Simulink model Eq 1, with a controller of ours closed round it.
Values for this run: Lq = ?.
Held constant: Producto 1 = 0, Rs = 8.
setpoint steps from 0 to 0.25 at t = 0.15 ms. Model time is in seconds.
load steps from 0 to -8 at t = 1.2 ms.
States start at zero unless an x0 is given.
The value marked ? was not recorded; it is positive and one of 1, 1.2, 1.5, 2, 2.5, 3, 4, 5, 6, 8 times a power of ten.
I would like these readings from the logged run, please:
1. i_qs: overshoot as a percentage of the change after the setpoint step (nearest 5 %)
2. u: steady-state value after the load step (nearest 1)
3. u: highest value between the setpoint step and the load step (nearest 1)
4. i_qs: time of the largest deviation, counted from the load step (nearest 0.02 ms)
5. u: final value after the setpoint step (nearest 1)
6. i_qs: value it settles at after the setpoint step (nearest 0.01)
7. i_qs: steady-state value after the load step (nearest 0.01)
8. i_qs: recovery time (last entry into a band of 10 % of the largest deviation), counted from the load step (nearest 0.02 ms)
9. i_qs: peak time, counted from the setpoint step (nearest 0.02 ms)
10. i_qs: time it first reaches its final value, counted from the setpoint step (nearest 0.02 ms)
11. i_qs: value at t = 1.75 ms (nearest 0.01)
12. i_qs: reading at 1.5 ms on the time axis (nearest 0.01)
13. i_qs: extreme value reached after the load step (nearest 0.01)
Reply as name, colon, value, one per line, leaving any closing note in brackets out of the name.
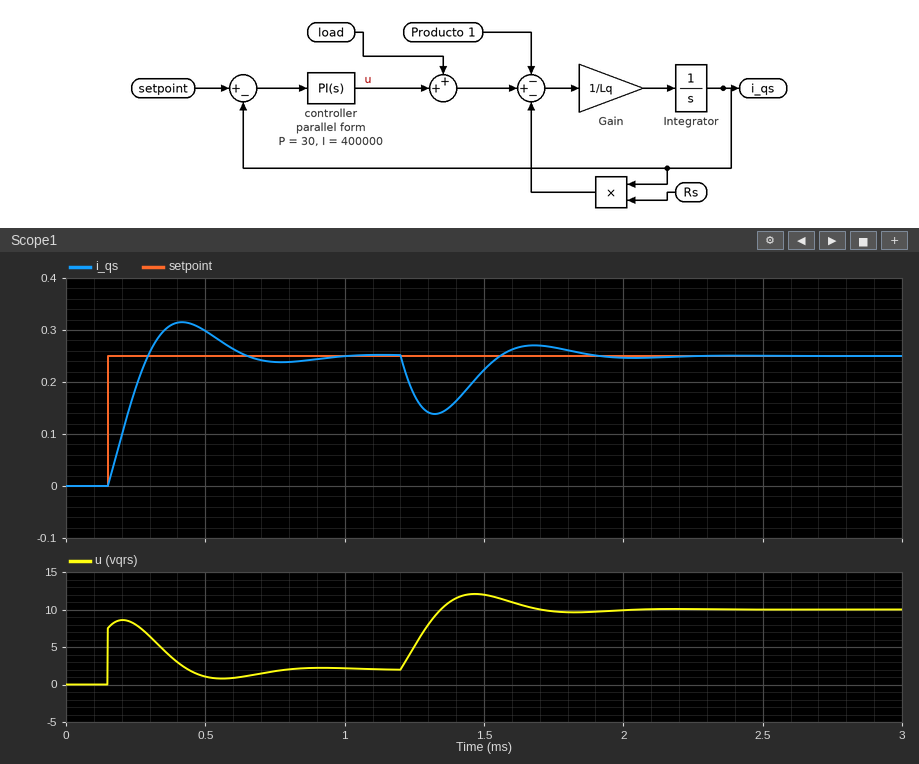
i_qs: overshoot as a percentage of the change after the setpoint step: 25 %
u: steady-state value after the load step: 10
u: highest value between the setpoint step and the load step: 9
i_qs: time of the largest deviation, counted from the load step: 0.12 ms
u: final value after the setpoint step: 2
i_qs: value it settles at after the setpoint step: 0.25
i_qs: steady-state value after the load step: 0.25
i_qs: recovery time (last entry into a band of 10 % of the largest deviation), counted from the load step: 0.60 ms
i_qs: peak time, counted from the setpoint step: 0.26 ms
i_qs: time it first reaches its final value, counted from the setpoint step: 0.14 ms
i_qs: value at t = 1.75 ms: 0.27
i_qs: reading at 1.5 ms on the time axis: 0.22
i_qs: extreme value reached after the load step: 0.14
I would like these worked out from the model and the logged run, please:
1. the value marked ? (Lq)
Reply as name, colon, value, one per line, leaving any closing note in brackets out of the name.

the value marked ?: 0.004
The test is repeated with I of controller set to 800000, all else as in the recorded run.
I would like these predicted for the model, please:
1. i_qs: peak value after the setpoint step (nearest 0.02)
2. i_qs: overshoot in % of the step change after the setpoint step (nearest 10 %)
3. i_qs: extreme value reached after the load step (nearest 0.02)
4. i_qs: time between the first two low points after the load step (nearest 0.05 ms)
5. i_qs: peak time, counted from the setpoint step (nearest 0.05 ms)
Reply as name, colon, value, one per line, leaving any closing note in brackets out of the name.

i_qs: peak value after the setpoint step: 0.34
i_qs: overshoot in % of the step change after the setpoint step: 40 %
i_qs: extreme value reached after the load step: 0.16
i_qs: time between the first two low points after the load step: 0.45 ms
i_qs: peak time, counted from the setpoint step: 0.20 ms
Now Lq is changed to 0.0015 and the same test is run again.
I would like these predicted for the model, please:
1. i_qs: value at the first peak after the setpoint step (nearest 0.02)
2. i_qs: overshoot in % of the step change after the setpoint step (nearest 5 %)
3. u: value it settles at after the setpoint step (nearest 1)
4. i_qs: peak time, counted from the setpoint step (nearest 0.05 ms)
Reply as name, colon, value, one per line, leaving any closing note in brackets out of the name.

i_qs: value at the first peak after the setpoint step: 0.28
i_qs: overshoot in % of the step change after the setpoint step: 10 %
u: value it settles at after the setpoint step: 2
i_qs: peak time, counted from the setpoint step: 0.15 ms
